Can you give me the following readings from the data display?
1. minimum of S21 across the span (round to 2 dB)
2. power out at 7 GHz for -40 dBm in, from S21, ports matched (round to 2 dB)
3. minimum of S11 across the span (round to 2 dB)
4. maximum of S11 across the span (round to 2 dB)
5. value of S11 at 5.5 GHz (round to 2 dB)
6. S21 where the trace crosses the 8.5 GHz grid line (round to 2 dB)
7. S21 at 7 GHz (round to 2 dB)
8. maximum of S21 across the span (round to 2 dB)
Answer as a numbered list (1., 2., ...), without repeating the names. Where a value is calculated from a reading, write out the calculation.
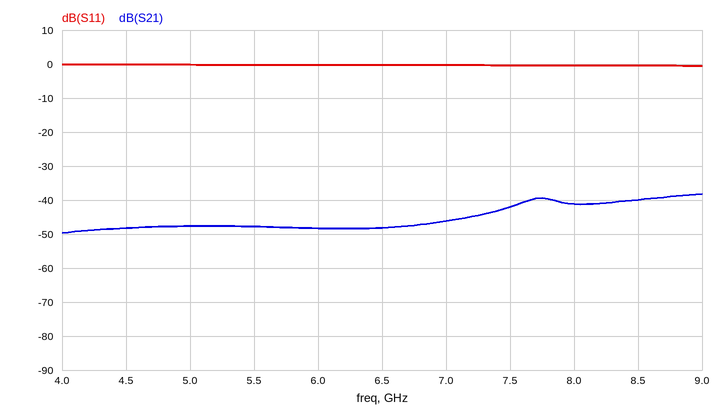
1. -50 dB
2. -40 dBm + (-46 dB) = -86 dBm
3. 0 dB
4. 0 dB
5. 0 dB
6. -40 dB
7. -46 dB
8. -38 dB
